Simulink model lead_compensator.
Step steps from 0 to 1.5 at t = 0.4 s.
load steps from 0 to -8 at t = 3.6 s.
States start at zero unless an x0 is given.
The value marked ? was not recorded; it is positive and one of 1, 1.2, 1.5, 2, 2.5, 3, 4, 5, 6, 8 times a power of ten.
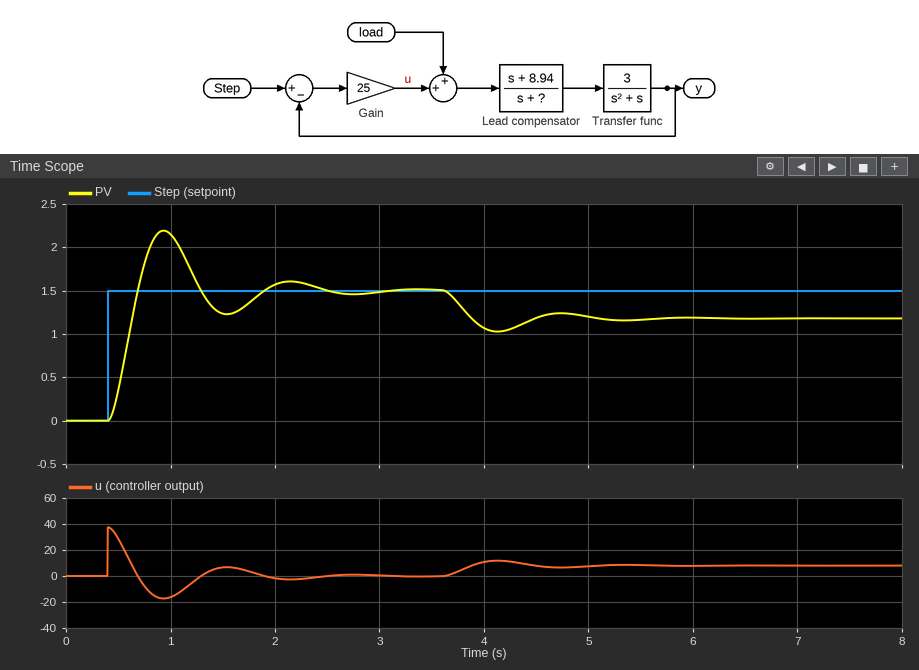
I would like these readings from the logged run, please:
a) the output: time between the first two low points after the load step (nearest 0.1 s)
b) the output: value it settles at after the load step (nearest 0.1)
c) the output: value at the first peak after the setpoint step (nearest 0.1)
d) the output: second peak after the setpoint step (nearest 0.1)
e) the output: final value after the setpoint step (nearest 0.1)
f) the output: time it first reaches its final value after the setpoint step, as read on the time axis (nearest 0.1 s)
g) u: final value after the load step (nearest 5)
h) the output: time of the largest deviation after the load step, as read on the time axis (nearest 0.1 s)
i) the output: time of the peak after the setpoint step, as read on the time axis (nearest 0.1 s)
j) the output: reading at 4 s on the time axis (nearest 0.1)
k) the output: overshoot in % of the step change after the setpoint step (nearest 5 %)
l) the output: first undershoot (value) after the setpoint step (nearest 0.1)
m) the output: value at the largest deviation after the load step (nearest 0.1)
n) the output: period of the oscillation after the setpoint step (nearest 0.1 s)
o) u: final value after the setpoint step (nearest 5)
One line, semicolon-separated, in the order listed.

1.2 s; 1.2; 2.2; 1.6; 1.5; 0.7 s; 10; 4.1 s; 0.9 s; 1.1; 45 %; 1.2; 1.0; 1.2 s; 0
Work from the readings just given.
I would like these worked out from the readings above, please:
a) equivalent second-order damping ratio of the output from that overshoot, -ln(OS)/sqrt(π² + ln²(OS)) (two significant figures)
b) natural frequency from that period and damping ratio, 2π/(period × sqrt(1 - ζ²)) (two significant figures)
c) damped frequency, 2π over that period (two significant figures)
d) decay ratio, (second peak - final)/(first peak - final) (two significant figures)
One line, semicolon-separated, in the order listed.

0.25; 5.4 rad/s; 5.2 rad/s; 0.14
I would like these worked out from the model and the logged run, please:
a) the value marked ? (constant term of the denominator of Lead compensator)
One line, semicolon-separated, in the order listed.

25
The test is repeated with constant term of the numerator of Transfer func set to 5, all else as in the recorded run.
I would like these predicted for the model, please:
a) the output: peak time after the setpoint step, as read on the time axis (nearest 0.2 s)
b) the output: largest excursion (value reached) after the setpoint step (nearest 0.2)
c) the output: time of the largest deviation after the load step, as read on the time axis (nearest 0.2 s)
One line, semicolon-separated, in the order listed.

0.8 s; 2.2; 4.0 s
